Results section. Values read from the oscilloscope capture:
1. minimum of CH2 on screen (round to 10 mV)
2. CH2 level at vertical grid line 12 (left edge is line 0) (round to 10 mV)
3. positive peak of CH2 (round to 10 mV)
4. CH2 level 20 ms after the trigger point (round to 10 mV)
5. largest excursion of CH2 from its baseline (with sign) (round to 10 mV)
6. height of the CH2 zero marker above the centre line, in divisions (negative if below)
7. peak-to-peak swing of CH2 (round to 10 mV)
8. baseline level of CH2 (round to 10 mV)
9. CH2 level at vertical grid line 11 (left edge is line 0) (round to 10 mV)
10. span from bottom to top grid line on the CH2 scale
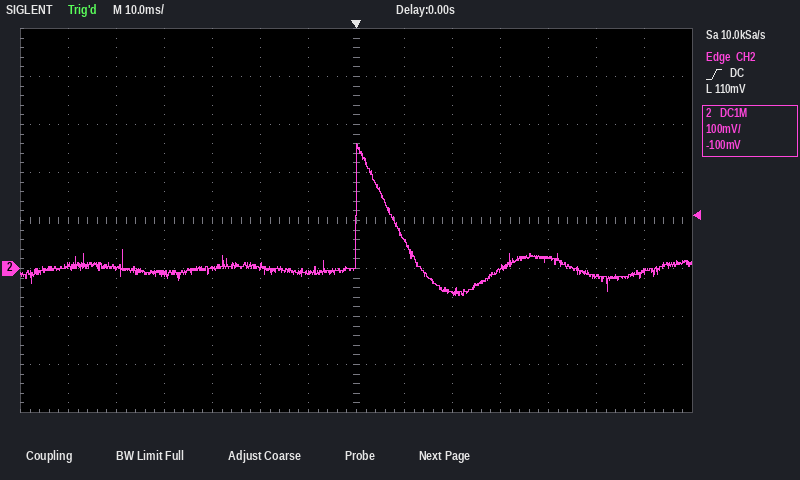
-60 mV
-20 mV
260 mV
-50 mV
+260 mV
-1.0 div
320 mV
0 mV
20 mV
800 mV
